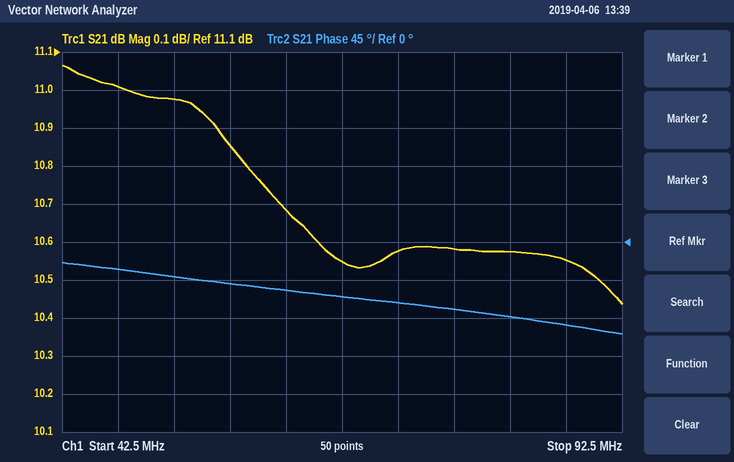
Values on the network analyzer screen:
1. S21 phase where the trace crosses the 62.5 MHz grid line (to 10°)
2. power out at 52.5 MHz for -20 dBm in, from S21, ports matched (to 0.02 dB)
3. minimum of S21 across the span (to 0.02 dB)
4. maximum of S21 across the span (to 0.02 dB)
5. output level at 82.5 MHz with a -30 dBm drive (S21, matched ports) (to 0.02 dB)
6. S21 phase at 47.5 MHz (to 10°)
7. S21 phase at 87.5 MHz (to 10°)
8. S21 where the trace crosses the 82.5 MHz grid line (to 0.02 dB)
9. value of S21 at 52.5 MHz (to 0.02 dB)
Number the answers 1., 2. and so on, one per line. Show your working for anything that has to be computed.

1. -60°
2. -20 dBm + (10.98 dB) = -9.02 dBm
3. 10.44 dB
4. 11.06 dB
5. -30 dBm + (10.58 dB) = -19.42 dBm
6. -30°
7. -100°
8. 10.58 dB
9. 10.98 dB
